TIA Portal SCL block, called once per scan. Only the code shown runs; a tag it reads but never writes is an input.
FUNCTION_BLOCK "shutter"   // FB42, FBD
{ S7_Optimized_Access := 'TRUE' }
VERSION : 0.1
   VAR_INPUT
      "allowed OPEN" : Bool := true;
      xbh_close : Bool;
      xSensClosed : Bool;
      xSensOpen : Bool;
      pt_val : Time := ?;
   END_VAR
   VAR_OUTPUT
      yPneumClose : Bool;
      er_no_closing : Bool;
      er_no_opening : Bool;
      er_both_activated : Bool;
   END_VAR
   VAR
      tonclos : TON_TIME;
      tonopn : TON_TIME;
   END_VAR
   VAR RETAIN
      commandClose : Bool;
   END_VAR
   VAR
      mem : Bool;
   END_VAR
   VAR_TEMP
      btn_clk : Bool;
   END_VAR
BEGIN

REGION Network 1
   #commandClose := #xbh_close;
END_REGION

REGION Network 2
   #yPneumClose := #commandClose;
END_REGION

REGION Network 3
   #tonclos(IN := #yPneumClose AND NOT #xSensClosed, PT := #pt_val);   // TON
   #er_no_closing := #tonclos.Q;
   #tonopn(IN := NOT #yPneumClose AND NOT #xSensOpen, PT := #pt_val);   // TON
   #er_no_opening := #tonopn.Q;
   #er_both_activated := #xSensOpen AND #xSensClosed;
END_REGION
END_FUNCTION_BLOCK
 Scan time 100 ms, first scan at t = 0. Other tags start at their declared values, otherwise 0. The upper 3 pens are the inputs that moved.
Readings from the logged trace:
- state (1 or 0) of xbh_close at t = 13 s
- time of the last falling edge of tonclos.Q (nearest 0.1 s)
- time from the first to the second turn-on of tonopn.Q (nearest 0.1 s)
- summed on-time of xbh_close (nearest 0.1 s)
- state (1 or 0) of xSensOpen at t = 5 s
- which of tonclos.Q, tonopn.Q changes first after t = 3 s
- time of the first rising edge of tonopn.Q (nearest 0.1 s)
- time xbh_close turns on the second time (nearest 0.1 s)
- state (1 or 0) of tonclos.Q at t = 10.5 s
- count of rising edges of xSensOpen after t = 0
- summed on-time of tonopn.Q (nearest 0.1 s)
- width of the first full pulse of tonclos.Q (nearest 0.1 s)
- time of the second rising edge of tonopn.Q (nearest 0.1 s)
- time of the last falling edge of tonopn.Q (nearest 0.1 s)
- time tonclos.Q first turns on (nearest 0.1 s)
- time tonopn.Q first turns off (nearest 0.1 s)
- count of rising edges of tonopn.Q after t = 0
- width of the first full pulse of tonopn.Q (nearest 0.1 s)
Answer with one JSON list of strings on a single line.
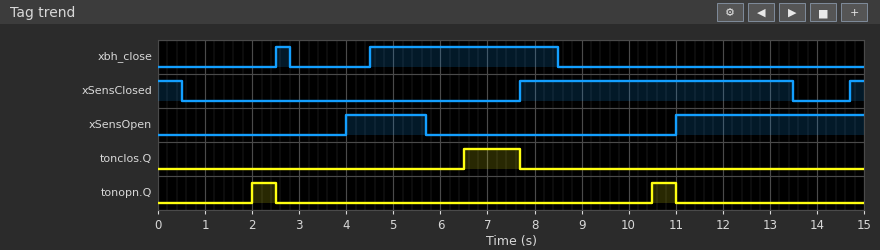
["0", "7.7 s", "8.5 s", "4.3 s", "1", "tonclos.Q", "2.0 s", "4.5 s", "0", "2", "1.0 s", "1.2 s", "10.5 s", "11.0 s", "6.5 s", "2.5 s", "2", "0.5 s"]
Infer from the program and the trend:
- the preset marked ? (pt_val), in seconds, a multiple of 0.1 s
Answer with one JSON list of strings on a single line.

["2.0 s"]
